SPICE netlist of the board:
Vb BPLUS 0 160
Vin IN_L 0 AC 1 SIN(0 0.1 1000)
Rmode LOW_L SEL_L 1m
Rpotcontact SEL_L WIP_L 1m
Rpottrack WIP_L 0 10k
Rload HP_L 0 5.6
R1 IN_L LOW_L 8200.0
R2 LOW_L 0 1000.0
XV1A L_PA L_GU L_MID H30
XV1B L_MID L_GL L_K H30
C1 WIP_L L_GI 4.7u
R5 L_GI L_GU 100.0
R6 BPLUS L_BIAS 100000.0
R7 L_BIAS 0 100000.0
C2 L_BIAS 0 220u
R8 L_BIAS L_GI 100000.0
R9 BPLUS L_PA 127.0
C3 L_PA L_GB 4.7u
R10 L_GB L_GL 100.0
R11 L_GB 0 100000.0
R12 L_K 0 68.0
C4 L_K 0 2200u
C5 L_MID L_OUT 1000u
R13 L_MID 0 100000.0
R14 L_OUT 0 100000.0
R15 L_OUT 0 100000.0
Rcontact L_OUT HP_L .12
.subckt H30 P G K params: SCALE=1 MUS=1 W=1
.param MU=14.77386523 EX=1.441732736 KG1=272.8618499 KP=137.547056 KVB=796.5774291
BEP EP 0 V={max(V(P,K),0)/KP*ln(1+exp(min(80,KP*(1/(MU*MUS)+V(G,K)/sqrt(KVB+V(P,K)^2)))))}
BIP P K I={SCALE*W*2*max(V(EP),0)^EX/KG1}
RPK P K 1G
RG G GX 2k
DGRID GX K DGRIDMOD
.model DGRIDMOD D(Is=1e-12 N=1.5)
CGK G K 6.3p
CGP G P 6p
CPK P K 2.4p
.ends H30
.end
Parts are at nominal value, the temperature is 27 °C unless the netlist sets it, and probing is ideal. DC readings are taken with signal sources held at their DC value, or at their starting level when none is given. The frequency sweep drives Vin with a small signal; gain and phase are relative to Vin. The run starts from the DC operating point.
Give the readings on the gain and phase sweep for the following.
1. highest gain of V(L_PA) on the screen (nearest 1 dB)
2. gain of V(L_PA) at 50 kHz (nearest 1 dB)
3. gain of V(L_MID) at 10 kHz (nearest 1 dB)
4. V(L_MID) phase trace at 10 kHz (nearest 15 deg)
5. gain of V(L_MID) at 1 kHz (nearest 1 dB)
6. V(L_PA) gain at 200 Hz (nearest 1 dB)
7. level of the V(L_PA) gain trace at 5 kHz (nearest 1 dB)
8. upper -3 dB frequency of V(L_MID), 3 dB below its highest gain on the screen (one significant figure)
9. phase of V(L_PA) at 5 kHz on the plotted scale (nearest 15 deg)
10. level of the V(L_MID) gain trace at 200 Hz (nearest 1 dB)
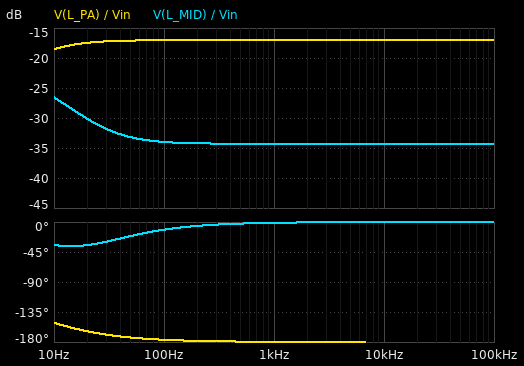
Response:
-17 dB
-17 dB
-34 dB
0 deg
-34 dB
-17 dB
-17 dB
20 Hz
-180 deg
-34 dB
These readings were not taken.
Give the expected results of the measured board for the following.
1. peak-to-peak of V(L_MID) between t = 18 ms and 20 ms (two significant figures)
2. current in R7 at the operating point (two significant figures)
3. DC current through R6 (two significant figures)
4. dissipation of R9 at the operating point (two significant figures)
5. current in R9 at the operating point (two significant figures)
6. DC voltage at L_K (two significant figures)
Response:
3.9 mV
800 µA
800 µA
180 mW
37 mA
2.5 V
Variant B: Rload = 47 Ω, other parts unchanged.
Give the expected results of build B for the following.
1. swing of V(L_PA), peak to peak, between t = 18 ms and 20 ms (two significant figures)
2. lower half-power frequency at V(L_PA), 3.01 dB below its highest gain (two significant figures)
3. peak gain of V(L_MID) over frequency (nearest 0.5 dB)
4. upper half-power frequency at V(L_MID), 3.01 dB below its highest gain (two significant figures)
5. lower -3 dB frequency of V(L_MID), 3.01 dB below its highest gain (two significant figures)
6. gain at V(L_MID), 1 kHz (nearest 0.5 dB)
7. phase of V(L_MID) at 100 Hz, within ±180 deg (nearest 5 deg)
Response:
12 mV
1.7 Hz
-22.5 dB
8.6 MHz
270 mHz
-24.0 dB
0 deg
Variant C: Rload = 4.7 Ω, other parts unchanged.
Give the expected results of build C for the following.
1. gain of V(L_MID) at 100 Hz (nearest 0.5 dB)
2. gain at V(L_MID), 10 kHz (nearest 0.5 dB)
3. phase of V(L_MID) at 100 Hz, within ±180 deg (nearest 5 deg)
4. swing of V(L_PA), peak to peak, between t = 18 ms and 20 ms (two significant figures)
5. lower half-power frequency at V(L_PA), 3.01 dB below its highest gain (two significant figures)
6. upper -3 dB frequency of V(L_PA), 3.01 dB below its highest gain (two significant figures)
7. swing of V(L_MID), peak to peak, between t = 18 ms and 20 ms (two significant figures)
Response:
-35.0 dB
-35.5 dB
-15 deg
29 mV
6.6 Hz
8.2 MHz
3.4 mV
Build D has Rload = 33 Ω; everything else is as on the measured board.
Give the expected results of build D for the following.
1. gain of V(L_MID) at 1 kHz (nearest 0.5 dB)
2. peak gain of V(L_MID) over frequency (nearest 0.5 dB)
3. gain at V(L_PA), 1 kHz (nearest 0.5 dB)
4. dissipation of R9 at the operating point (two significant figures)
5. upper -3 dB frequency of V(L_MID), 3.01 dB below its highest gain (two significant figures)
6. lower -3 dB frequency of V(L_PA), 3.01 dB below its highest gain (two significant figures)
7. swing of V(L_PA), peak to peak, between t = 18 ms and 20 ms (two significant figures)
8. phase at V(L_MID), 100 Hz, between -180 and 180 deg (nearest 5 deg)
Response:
-25.0 dB
-22.5 dB
-23.0 dB
180 mW
2.5 MHz
2.5 Hz
14 mV
0 deg
